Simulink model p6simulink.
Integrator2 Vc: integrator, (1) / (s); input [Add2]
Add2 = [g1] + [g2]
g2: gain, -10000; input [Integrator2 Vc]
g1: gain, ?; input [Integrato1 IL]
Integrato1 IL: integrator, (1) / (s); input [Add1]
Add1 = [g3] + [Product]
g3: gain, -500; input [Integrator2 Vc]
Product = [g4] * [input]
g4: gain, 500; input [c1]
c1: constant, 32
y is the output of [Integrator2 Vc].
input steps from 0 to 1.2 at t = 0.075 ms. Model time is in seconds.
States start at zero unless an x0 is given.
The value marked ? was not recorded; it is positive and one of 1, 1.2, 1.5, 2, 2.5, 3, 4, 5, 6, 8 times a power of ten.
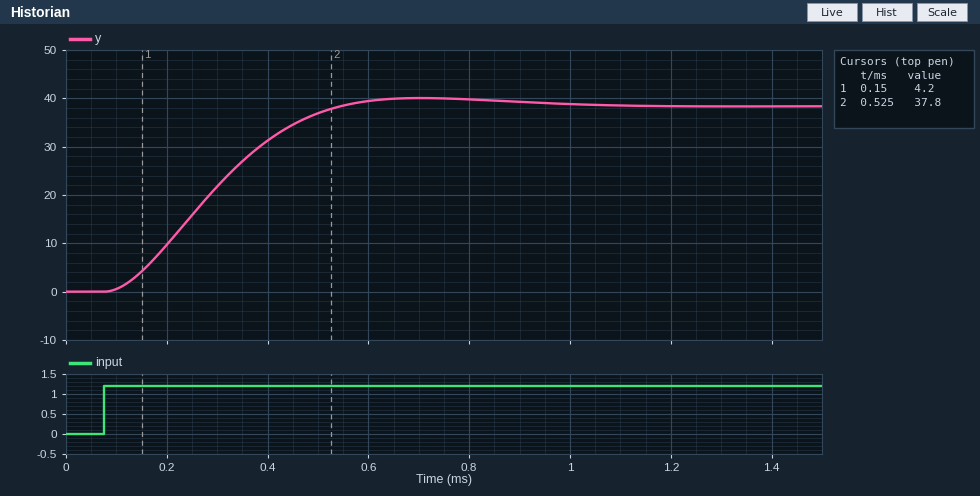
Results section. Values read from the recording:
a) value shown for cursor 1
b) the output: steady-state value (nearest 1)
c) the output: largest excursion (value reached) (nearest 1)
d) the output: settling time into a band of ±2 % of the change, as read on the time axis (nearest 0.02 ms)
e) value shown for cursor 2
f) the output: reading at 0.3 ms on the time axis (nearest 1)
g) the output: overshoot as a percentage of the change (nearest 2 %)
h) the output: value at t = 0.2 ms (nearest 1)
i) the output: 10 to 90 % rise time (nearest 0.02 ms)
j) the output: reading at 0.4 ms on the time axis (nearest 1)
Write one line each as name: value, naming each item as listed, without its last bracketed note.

value shown for cursor 1: 4.2
the output: steady-state value: 38
the output: largest excursion (value reached): 40
the output: settling time into a band of ±2 % of the change, as read on the time axis: 0.92 ms
value shown for cursor 2: 37.8
the output: reading at 0.3 ms on the time axis: 22
the output: overshoot as a percentage of the change: 4 %
the output: value at t = 0.2 ms: 10
the output: 10 to 90 % rise time: 0.30 ms
the output: reading at 0.4 ms on the time axis: 31
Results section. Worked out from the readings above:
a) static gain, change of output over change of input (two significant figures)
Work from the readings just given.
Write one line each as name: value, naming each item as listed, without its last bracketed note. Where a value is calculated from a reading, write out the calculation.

static gain, change of output over change of input: (38 - 0) / (1.2 - 0) = 32
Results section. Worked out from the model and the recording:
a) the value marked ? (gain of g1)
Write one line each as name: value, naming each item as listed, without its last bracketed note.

the value marked ?: 100000
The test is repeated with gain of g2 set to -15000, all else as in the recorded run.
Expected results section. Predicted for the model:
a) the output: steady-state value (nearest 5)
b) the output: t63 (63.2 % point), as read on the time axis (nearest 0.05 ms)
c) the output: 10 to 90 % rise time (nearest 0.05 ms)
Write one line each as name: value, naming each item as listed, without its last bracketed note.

the output: steady-state value: 40
the output: t63 (63.2 % point), as read on the time axis: 0.40 ms
the output: 10 to 90 % rise time: 0.50 ms
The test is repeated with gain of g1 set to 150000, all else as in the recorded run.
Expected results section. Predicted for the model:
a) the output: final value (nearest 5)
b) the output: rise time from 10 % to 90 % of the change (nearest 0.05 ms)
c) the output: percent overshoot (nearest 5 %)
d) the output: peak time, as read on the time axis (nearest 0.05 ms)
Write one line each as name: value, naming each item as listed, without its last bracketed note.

the output: final value: 40
the output: rise time from 10 % to 90 % of the change: 0.20 ms
the output: percent overshoot: 10 %
the output: peak time, as read on the time axis: 0.50 ms
